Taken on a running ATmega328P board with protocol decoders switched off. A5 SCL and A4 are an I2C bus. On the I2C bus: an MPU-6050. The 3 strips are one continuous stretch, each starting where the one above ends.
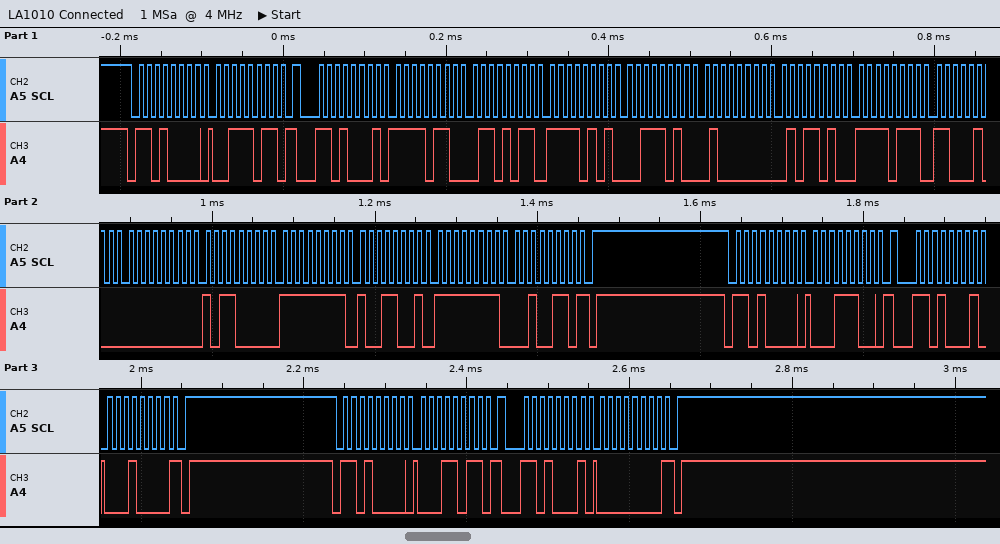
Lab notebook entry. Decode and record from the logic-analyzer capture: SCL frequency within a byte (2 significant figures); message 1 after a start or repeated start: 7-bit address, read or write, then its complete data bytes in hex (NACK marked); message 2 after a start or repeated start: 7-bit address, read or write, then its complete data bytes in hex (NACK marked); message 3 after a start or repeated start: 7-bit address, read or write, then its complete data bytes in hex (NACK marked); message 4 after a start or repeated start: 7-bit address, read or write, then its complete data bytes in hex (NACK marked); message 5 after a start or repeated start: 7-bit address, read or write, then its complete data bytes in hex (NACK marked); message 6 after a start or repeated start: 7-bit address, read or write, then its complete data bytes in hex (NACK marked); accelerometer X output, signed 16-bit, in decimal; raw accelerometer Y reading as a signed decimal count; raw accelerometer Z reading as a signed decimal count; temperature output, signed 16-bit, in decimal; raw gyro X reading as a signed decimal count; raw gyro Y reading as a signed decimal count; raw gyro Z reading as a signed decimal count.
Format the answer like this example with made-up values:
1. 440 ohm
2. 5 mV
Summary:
1. 100 kHz
2. 0x68 write: 3B
3. 0x68 read: F6 6B F5 3A 40 5A F7 C4 00 B0 FF 99 FF 26 NACK
4. 0x68 write: 1C
5. 0x68 read: 10 NACK
6. 0x68 write: 1B
7. 0x68 read: 00 NACK
8. -2453
9. -2758
10. 16474
11. -2108
12. 176
13. -103
14. -218
